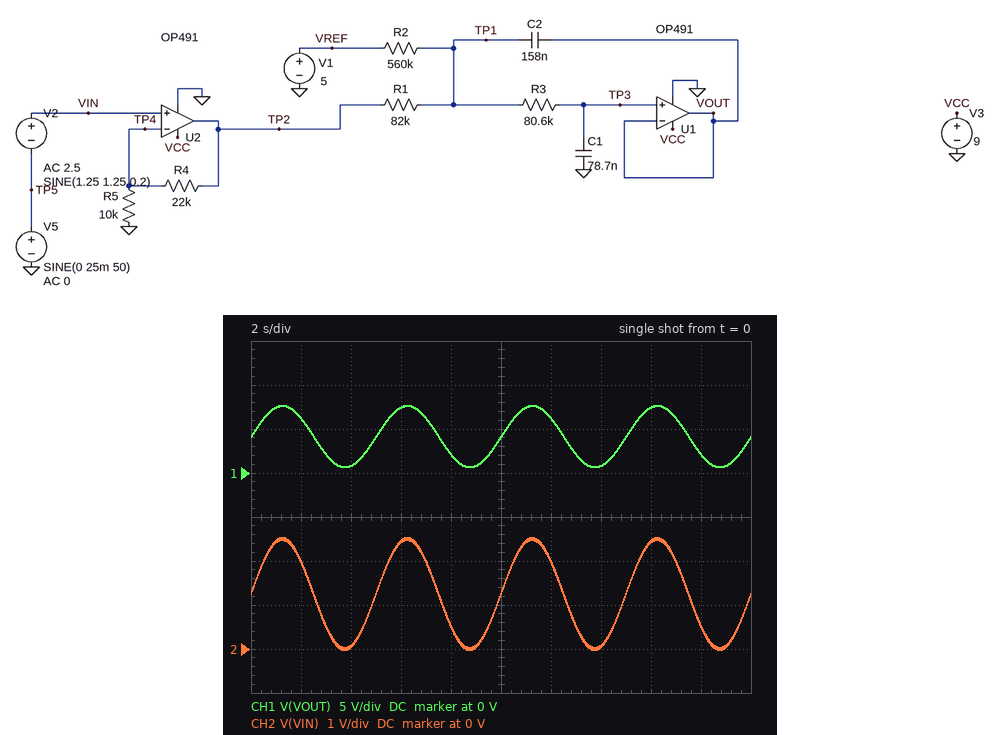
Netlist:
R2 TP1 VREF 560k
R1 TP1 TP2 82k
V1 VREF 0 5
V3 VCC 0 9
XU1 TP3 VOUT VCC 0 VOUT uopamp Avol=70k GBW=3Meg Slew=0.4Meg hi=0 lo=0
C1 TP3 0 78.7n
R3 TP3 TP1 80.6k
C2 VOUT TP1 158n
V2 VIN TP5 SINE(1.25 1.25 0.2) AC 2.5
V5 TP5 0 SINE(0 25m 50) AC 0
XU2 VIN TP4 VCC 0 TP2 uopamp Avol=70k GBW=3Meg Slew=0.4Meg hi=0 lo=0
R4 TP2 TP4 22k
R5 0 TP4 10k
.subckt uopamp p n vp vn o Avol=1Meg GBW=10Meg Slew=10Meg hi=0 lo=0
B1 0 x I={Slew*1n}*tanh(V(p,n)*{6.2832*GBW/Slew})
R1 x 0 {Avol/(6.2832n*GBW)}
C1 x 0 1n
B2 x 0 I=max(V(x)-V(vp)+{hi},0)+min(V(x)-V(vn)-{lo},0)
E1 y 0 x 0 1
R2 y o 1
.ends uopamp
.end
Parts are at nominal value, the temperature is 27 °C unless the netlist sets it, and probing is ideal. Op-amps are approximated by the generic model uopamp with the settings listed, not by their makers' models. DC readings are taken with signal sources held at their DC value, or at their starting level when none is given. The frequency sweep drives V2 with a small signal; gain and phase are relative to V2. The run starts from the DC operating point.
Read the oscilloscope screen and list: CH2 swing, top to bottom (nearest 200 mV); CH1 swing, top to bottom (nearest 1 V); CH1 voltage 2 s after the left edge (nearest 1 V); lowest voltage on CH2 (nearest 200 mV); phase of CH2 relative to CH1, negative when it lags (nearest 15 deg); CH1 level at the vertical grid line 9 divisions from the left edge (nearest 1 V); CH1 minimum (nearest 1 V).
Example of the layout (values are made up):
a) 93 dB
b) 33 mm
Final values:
a) 2.6 V
b) 7 V
c) 6 V
d) 0 V
e) 0 deg
f) 2 V
g) 1 V
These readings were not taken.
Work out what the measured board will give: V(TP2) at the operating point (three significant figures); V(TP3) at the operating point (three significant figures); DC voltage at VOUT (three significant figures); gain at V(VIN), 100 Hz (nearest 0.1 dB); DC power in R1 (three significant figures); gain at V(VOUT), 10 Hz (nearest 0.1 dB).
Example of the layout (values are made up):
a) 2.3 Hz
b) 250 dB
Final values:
a) 4.00 V
b) 4.13 V
c) 4.13 V
d) 0 dB
e) 199 nW
f) 8.6 dB
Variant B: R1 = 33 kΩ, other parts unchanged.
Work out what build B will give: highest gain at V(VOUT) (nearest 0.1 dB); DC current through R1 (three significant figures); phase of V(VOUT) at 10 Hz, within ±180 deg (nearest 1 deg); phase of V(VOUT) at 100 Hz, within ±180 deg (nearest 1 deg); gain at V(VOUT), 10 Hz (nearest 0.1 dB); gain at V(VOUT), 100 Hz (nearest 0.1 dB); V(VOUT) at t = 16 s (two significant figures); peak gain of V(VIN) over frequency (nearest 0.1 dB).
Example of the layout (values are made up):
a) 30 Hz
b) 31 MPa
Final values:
a) 9.6 dB
b) 1.69 µA
c) -32 deg
d) -154 deg
e) 9.3 dB
f) -12.4 dB
g) 7.6 V
h) 0 dB
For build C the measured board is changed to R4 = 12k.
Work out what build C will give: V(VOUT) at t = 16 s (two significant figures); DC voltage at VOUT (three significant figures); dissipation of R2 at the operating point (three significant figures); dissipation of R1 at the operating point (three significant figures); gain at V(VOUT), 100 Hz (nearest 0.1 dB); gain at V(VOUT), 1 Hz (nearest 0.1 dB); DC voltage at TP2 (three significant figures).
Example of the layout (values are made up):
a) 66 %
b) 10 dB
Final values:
a) 5.3 V
b) 3.04 V
c) 6.88 µW
d) 1.01 µW
e) -23.4 dB
f) 5.7 dB
g) 2.75 V
